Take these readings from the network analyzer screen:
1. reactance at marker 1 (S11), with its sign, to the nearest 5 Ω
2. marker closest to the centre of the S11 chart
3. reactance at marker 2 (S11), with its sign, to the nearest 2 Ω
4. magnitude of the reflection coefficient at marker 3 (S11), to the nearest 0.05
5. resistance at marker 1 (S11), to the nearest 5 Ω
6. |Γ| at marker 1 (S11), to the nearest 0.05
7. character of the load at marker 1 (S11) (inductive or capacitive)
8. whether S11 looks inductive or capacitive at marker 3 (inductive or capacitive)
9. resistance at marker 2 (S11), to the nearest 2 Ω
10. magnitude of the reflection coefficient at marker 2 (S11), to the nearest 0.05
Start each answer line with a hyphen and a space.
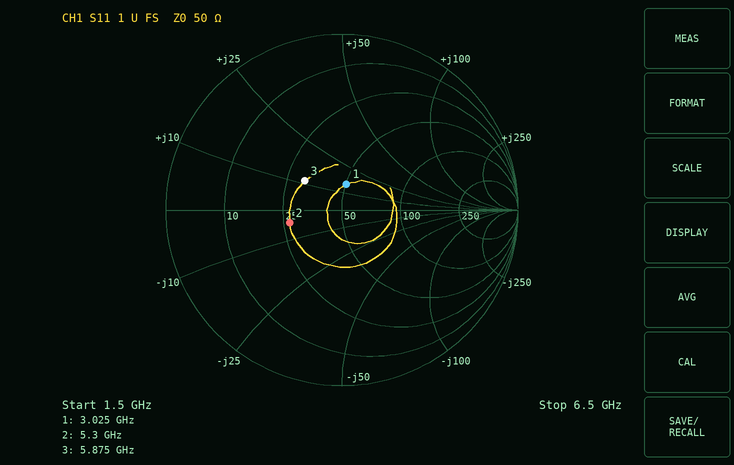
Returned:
- +15 Ω
- marker 1
- -4 Ω
- 0.25
- 50 Ω
- 0.15
- inductive
- inductive
- 26 Ω
- 0.30
